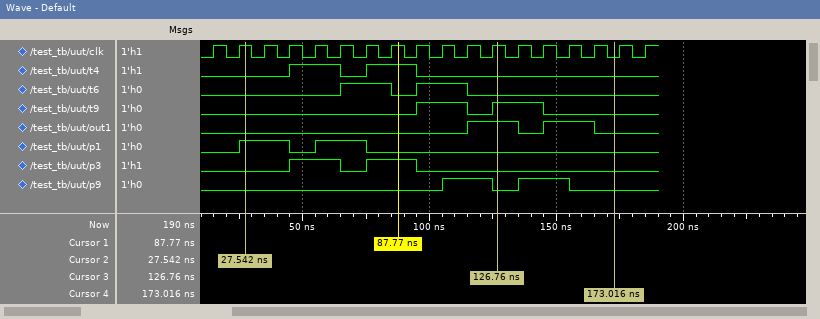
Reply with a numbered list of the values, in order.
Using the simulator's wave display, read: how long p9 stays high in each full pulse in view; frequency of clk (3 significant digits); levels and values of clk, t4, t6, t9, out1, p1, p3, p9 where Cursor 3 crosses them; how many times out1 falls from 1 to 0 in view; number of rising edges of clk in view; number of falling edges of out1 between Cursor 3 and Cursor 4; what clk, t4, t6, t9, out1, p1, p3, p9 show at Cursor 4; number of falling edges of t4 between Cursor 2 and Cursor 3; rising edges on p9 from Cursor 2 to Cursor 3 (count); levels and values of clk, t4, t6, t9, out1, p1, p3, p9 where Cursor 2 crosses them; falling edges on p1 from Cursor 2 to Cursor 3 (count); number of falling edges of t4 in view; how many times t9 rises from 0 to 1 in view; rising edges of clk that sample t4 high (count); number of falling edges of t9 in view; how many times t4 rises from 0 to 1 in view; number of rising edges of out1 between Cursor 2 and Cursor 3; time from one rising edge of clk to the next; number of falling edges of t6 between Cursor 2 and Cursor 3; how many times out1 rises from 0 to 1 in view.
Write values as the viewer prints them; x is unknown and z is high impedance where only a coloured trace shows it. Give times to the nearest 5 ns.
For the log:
1. 20 ns, 20 ns
2. 100 MHz
3. clk=1, t4=0, t6=0, t9=1, out1=1, p1=0, p3=0, p9=0
4. 2
5. 18
6. 2
7. clk=0, t4=0, t6=0, t9=0, out1=0, p1=0, p3=0, p9=0
8. 2
9. 1
10. clk=1, t4=0, t6=0, t9=0, out1=0, p1=1, p3=0, p9=0
11. 2
12. 2
13. 2
14. 4
15. 2
16. 2
17. 1
18. 10 ns
19. 2
20. 2
